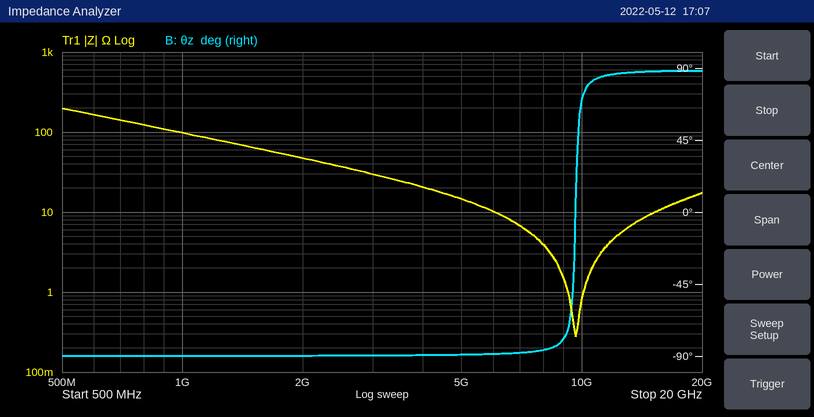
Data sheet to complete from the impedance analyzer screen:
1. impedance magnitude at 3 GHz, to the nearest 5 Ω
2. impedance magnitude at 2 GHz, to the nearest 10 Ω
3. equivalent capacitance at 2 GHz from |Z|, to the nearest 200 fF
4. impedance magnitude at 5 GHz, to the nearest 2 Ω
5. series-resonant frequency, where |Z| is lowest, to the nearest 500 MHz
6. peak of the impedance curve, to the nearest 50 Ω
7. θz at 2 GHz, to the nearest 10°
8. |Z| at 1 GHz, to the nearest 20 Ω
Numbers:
30 Ω
50 Ω
1.6 pF
14 Ω
9.5 GHz
200 Ω
-90°
100 Ω
